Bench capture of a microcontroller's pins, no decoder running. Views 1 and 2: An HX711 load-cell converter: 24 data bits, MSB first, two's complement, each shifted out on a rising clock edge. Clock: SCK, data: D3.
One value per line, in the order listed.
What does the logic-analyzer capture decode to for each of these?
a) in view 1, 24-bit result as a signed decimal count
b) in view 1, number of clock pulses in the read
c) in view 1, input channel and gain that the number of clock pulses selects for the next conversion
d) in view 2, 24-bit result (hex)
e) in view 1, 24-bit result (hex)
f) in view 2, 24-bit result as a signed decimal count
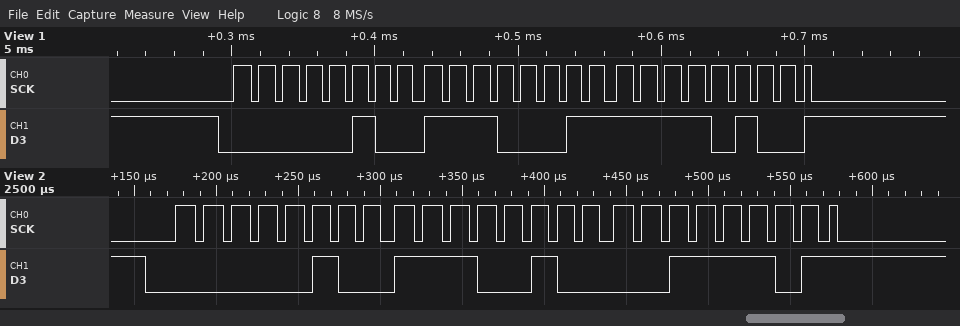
320500
25
channel A, gain 128
0x04E43D
0x04E3F4
320573
